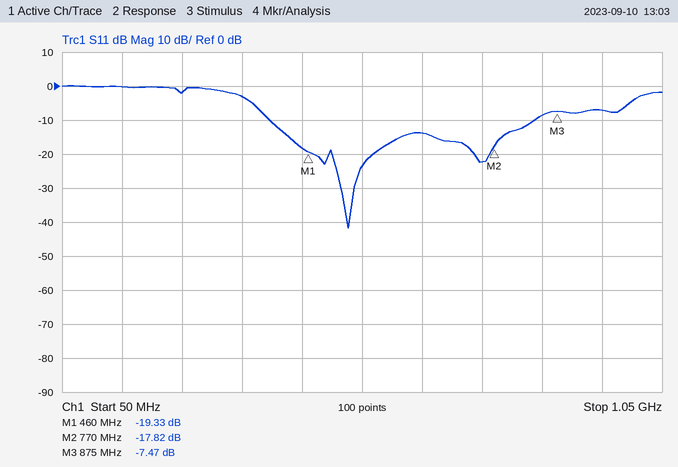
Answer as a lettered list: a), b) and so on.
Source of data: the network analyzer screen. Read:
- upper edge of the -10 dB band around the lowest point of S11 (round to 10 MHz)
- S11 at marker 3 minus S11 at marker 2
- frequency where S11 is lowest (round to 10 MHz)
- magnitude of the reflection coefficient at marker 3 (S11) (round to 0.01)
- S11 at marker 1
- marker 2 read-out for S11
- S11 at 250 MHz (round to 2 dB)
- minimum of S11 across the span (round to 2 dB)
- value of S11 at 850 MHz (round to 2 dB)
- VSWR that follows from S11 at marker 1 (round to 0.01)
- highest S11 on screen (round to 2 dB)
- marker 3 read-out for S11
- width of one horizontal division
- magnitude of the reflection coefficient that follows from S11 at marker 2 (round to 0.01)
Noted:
a) 840 MHz
b) 10.35 dB
c) 530 MHz
d) 0.42
e) -19.33 dB
f) -17.82 dB
g) -2 dB
h) -42 dB
i) -8 dB
j) 1.24
k) 0 dB
l) -7.47 dB
m) 100 MHz
n) 0.13
